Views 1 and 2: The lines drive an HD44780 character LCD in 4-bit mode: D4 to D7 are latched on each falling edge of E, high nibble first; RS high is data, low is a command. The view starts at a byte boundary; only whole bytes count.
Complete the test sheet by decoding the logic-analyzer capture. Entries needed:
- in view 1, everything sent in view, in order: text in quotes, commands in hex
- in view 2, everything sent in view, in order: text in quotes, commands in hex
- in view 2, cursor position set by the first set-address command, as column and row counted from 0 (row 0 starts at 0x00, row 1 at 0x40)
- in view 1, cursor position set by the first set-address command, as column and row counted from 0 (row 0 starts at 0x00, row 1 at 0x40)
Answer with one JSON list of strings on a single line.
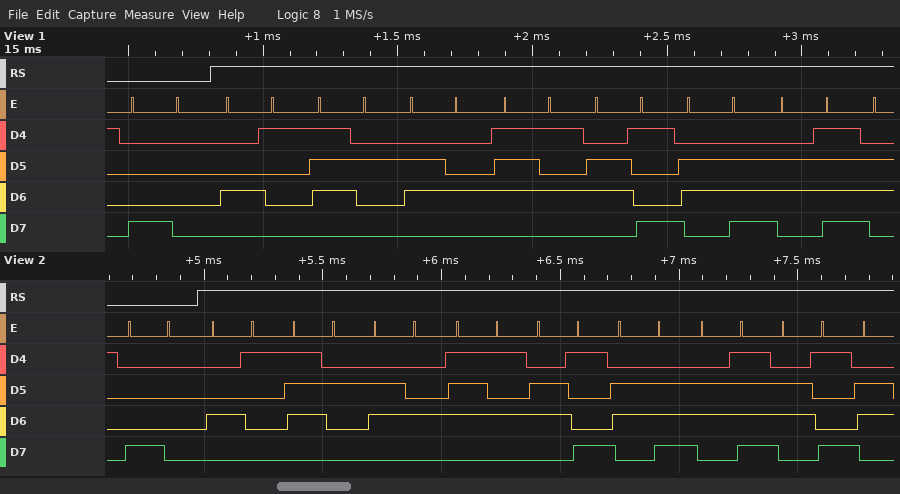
["0x80 \"Arduino\"", "0x80 \"Arduinoi\"", "column 0, row 0", "column 0, row 0"]
